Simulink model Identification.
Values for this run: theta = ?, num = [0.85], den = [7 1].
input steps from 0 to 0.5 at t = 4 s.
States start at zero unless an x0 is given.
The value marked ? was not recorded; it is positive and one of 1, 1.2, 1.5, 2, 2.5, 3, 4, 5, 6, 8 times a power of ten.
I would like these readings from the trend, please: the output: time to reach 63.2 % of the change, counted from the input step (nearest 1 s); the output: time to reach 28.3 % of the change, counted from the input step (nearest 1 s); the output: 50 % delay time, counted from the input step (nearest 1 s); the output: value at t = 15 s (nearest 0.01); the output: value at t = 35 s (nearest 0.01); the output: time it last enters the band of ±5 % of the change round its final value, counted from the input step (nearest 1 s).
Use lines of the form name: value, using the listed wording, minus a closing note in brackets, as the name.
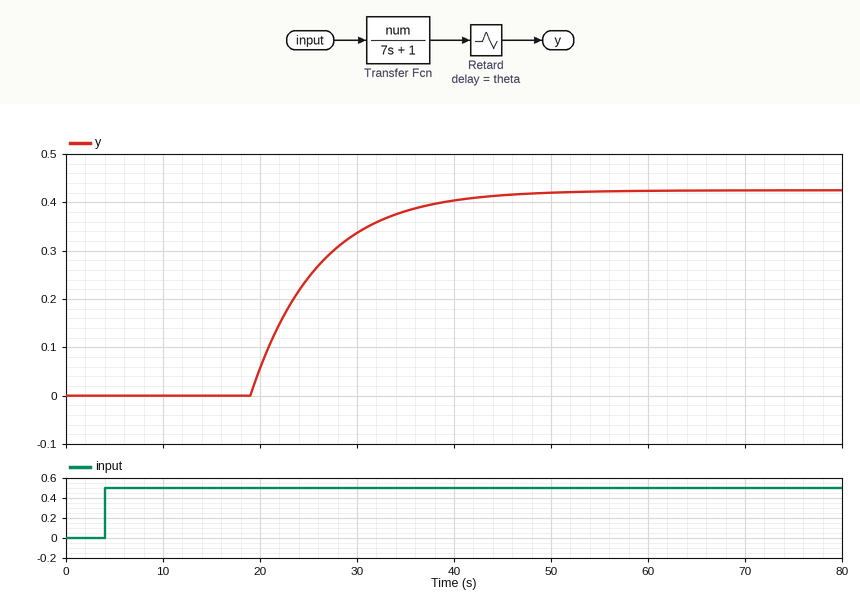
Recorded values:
the output: time to reach 63.2 % of the change, counted from the input step: 22 s
the output: time to reach 28.3 % of the change, counted from the input step: 17 s
the output: 50 % delay time, counted from the input step: 20 s
the output: value at t = 15 s: 0.00
the output: value at t = 35 s: 0.38
the output: time it last enters the band of ±5 % of the change round its final value, counted from the input step: 36 s
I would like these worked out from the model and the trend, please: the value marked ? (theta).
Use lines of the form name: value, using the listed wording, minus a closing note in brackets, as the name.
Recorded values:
the value marked ?: 15
